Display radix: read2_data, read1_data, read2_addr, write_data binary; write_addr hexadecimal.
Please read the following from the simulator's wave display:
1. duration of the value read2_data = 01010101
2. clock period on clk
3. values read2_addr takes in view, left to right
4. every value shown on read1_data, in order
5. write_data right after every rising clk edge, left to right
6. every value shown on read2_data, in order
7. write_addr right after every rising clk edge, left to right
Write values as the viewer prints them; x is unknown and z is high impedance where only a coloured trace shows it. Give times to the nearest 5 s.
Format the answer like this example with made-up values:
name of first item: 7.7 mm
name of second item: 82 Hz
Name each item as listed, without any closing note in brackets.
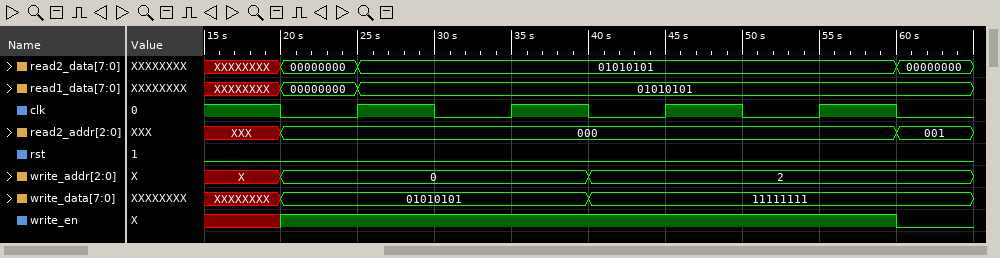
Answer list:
duration of the value read2_data = 01010101: 35 s
clock period on clk: 10 s
values read2_addr takes in view, left to right: XXX, 000, 001
every value shown on read1_data, in order: XXXXXXXX, 00000000, 01010101
write_data right after every rising clk edge, left to right: 01010101, 01010101, 11111111, 11111111
every value shown on read2_data, in order: XXXXXXXX, 00000000, 01010101, 00000000
write_addr right after every rising clk edge, left to right: 0, 0, 2, 2
